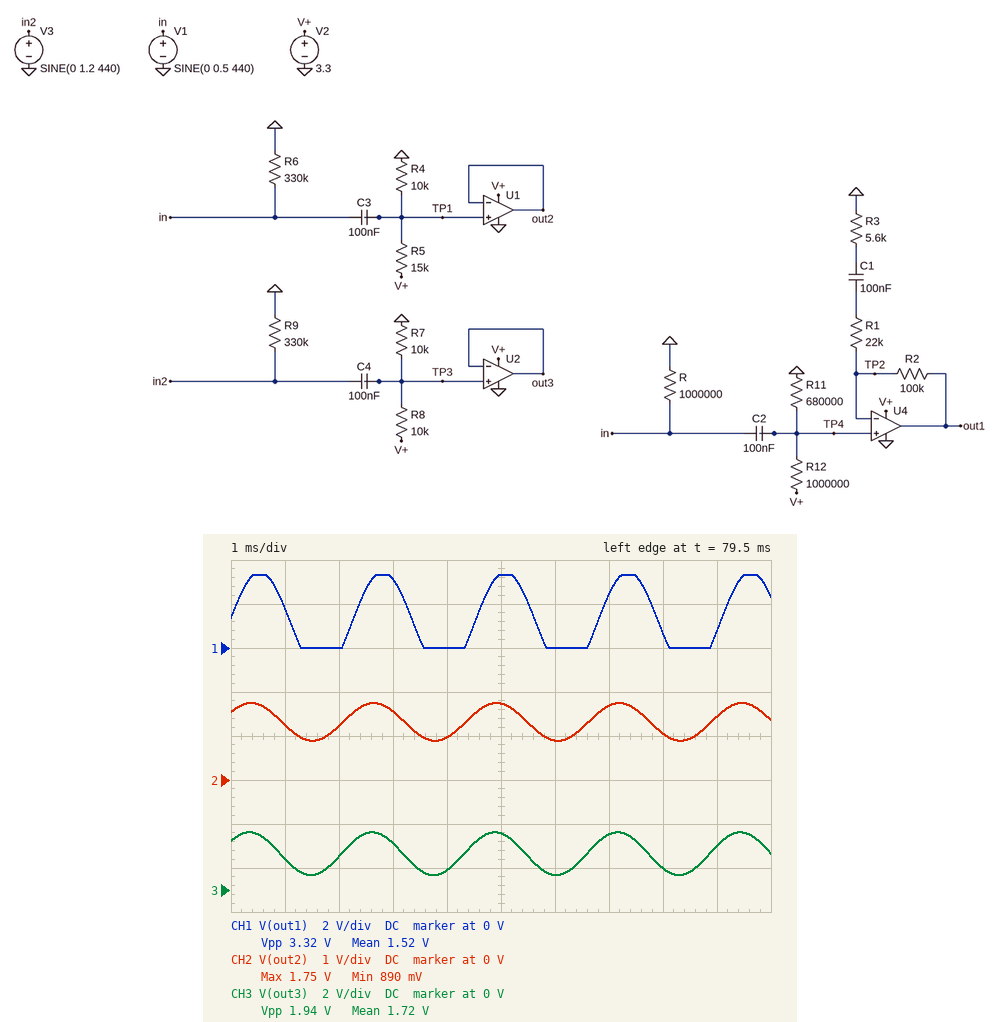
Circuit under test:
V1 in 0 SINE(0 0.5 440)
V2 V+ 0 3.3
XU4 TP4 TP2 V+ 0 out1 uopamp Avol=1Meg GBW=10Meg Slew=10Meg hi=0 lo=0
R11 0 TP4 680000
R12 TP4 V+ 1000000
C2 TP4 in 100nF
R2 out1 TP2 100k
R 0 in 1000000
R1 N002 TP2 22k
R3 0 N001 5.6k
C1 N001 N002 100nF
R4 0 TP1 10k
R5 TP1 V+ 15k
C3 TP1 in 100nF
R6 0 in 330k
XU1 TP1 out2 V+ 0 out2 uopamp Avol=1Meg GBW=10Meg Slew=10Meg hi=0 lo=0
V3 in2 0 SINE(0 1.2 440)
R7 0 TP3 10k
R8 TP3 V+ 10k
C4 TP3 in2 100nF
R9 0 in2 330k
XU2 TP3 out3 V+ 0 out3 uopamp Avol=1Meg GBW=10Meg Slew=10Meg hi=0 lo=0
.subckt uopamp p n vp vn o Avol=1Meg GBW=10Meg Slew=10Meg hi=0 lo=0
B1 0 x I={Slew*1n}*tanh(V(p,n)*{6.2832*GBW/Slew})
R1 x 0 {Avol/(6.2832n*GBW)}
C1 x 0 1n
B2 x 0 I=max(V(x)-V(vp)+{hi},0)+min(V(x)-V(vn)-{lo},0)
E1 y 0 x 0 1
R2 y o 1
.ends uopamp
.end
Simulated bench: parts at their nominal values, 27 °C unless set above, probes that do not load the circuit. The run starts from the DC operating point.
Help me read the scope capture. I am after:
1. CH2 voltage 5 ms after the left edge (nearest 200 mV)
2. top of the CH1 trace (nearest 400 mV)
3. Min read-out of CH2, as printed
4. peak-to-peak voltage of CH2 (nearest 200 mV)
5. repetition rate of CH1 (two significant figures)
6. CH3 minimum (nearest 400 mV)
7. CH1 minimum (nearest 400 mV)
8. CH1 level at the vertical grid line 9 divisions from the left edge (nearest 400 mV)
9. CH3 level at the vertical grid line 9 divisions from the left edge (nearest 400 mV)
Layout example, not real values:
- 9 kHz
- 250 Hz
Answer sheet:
- 1.8 V
- 3.2 V
- 890 mV
- 800 mV
- 440 Hz
- 800 mV
- 0 V
- 800 mV
- 2.0 V
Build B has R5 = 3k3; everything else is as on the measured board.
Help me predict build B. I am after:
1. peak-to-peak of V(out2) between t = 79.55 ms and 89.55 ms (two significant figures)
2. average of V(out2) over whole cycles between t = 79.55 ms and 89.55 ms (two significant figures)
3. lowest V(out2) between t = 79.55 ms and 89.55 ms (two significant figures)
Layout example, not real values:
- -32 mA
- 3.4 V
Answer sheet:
- 570 mV
- 2.5 V
- 2.2 V
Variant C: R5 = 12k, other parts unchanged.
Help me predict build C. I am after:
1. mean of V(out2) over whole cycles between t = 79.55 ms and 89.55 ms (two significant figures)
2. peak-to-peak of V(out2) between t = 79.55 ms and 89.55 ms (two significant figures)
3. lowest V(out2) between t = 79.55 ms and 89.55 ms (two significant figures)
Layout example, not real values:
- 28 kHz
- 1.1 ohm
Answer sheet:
- 1.5 V
- 830 mV
- 1.1 V
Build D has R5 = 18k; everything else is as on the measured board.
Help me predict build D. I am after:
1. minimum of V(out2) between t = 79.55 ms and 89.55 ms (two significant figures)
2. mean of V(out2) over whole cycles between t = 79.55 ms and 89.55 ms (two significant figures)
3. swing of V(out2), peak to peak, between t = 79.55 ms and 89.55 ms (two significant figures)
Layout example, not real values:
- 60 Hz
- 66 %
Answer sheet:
- 740 mV
- 1.2 V
- 870 mV
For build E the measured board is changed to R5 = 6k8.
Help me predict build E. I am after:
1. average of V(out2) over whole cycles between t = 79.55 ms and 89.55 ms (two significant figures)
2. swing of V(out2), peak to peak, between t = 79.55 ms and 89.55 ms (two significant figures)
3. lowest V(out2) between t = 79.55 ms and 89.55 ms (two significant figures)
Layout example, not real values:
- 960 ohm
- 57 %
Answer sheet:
- 2.0 V
- 750 mV
- 1.6 V
